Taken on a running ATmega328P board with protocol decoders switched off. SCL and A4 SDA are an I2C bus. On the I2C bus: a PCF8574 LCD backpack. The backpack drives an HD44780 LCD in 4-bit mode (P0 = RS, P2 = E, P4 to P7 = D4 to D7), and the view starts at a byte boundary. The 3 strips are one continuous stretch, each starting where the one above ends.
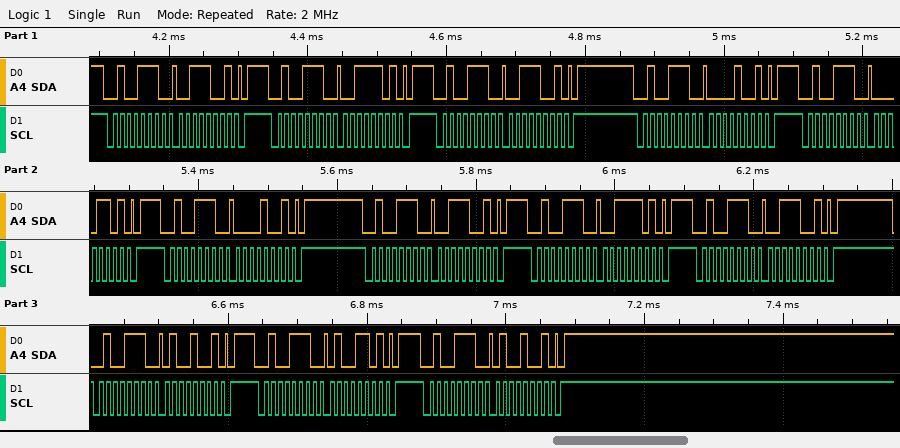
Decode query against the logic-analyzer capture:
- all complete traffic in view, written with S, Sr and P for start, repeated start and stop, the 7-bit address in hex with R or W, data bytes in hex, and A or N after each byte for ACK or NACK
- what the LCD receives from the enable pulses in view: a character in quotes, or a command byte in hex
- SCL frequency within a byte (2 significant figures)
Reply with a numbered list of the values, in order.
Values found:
1. S 27W A 39 A P S 27W A 3D A P S 27W A 39 A P S 27W A 09 A P S 27W A 0D A P S 27W A 09 A P S 27W A 39 A P S 27W A 3D A P S 27W A 39 A P S 27W A 49 A P S 27W A 4D A P S 27W A 49 A P
2. '0' '4'
3. 100 kHz
